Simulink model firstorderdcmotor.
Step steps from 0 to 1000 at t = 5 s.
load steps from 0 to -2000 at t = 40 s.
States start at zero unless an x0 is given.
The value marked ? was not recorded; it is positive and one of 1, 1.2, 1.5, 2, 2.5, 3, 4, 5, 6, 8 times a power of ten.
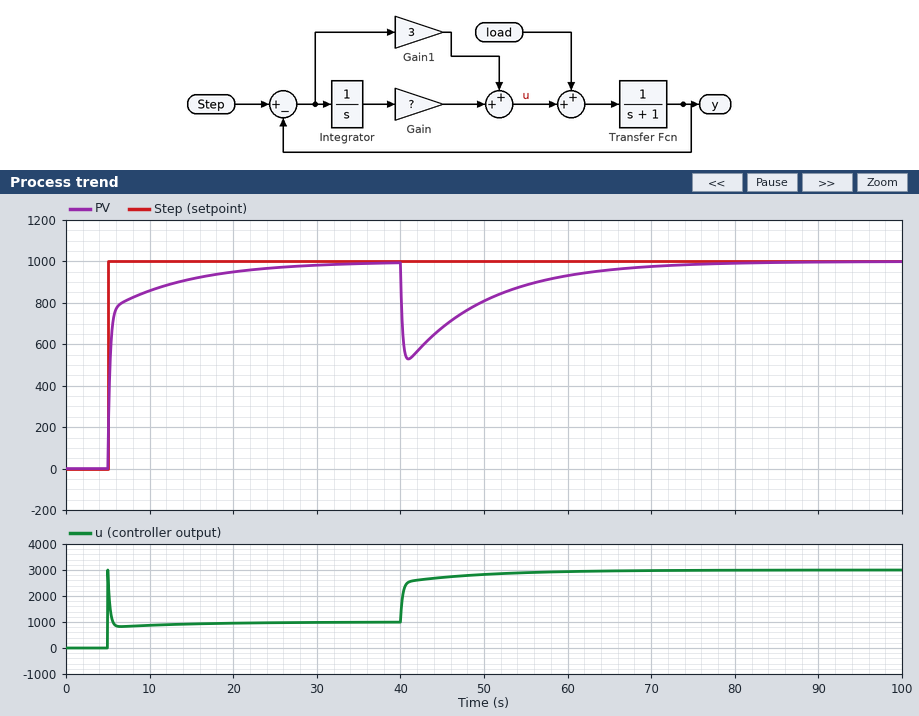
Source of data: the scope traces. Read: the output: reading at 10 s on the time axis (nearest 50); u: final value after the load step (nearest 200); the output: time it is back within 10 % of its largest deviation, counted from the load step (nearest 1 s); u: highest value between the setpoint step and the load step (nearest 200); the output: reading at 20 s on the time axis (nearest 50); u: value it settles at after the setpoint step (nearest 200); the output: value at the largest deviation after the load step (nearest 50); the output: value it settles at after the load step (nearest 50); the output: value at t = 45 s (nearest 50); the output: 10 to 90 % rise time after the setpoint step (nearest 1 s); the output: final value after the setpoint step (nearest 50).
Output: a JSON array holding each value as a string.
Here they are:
["850", "3000", "24 s", "3000", "950", "1000", "550", "1000", "700", "8 s", "1000"]
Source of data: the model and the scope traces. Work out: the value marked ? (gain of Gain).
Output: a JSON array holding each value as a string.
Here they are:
["0.4"]
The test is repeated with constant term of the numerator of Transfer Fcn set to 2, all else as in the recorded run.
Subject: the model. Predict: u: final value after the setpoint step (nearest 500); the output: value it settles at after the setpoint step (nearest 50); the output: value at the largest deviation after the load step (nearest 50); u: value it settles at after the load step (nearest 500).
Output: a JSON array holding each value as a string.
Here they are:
["500", "1000", "450", "2500"]
